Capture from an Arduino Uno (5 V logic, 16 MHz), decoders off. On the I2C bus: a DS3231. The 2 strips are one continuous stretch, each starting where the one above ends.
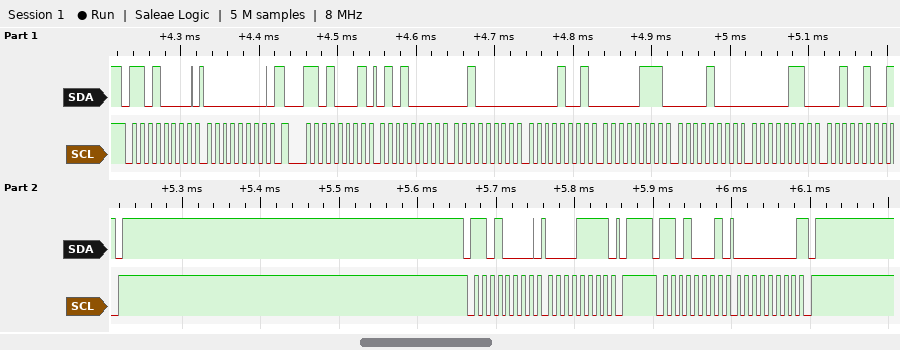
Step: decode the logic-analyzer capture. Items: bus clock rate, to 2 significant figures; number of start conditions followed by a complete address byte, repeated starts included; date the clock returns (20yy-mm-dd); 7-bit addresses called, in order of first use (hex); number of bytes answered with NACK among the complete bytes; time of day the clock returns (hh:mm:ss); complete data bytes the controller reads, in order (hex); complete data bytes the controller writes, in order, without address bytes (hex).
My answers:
100 kHz
4
2024-06-08
0x68
2
09:20:50
50 20 09 07 08 06 24 00
00 0F
